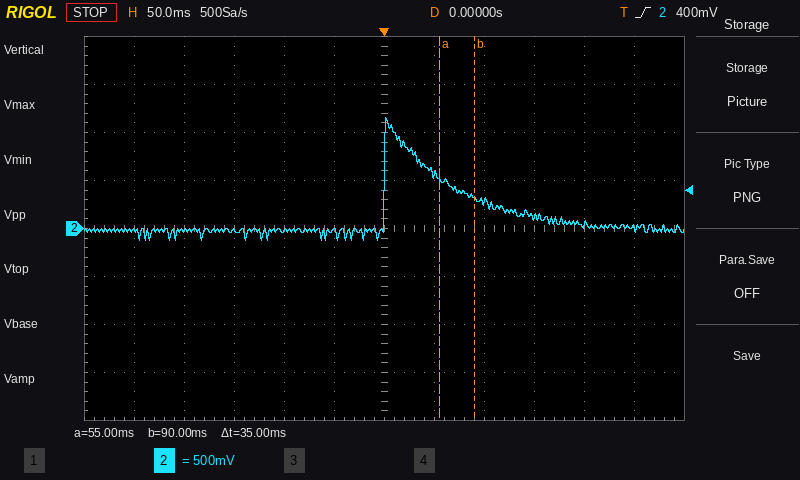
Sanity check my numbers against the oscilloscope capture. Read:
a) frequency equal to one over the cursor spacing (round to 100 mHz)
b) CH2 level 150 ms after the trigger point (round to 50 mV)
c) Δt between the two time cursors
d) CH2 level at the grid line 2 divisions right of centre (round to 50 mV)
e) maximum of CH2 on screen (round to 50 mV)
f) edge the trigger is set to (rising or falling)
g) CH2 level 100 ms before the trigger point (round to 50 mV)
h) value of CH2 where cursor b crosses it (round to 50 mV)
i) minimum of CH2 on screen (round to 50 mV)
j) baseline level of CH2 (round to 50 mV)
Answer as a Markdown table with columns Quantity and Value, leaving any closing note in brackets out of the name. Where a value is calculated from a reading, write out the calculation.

| Quantity | Value |
|---|---|
| frequency equal to one over the cursor spacing | 1 / 35 ms ≈ 28.6 Hz |
| CH2 level 150 ms after the trigger point | 100 mV |
| Δt between the two time cursors | 35 ms |
| CH2 level at the grid line 2 divisions right of centre | 300 mV |
| maximum of CH2 on screen | 1.15 V |
| edge the trigger is set to | rising |
| CH2 level 100 ms before the trigger point | 0 mV |
| value of CH2 where cursor b crosses it | 300 mV |
| minimum of CH2 on screen | -100 mV |
| baseline level of CH2 | 0 mV |
